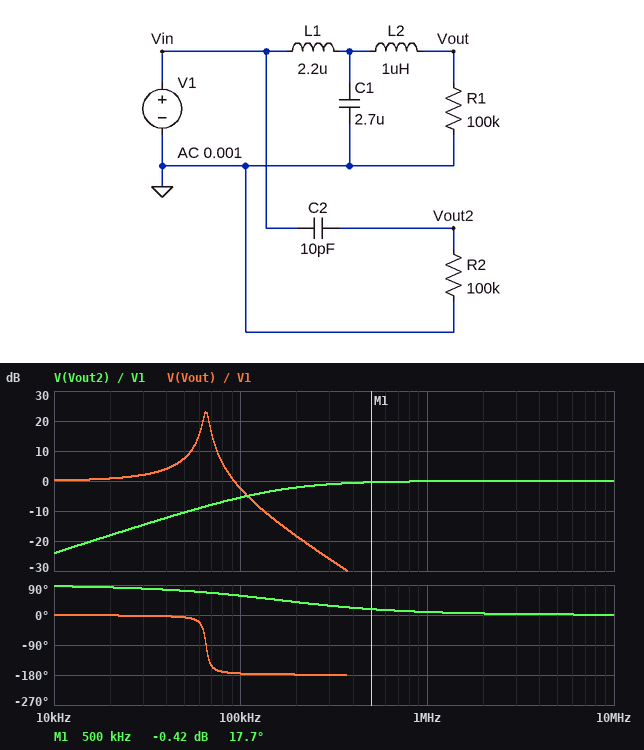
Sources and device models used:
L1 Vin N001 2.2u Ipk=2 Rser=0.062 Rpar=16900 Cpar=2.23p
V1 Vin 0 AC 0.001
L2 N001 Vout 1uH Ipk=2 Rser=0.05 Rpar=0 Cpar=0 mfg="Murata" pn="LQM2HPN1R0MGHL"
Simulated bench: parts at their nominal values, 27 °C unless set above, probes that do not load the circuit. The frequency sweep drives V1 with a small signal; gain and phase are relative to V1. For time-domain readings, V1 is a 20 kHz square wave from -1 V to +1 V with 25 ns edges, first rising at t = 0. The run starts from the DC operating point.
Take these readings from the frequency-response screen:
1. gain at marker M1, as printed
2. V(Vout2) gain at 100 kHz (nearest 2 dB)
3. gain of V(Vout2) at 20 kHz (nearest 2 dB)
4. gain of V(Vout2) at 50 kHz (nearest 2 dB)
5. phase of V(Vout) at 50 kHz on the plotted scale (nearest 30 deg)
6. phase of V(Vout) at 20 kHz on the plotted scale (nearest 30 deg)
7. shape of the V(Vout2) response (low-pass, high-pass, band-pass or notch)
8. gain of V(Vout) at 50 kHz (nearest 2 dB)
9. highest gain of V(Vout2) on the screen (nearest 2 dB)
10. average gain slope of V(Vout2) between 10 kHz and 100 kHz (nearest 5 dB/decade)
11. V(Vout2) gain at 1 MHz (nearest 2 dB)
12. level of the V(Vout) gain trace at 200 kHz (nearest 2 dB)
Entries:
-0.42 dB
-6 dB
-18 dB
-10 dB
0 deg
0 deg
high-pass
8 dB
0 dB
20 dB/decade
0 dB
-18 dB
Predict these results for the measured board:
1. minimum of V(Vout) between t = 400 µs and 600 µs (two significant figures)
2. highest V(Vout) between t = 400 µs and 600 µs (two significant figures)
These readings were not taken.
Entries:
-3.5 V
3.5 V
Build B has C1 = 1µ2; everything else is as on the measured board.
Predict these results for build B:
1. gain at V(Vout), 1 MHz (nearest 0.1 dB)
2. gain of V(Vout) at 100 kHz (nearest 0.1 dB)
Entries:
-40.3 dB
24.0 dB
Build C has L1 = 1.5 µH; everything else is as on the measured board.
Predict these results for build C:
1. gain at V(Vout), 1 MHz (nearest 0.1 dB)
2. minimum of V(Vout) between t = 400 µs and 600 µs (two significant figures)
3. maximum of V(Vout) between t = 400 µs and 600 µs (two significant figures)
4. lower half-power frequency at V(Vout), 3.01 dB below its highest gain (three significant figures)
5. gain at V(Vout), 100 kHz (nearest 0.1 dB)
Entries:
-44.0 dB
-2.1 V
2.1 V
75.6 kHz
4.3 dB
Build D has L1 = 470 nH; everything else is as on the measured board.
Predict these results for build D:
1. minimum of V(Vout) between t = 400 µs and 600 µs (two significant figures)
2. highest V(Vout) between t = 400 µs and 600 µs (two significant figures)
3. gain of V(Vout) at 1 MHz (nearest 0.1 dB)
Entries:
-3.0 V
3.0 V
-33.8 dB
